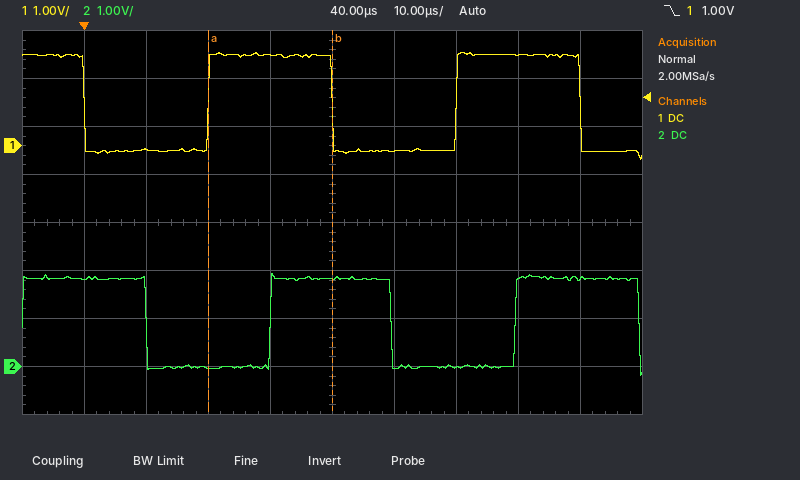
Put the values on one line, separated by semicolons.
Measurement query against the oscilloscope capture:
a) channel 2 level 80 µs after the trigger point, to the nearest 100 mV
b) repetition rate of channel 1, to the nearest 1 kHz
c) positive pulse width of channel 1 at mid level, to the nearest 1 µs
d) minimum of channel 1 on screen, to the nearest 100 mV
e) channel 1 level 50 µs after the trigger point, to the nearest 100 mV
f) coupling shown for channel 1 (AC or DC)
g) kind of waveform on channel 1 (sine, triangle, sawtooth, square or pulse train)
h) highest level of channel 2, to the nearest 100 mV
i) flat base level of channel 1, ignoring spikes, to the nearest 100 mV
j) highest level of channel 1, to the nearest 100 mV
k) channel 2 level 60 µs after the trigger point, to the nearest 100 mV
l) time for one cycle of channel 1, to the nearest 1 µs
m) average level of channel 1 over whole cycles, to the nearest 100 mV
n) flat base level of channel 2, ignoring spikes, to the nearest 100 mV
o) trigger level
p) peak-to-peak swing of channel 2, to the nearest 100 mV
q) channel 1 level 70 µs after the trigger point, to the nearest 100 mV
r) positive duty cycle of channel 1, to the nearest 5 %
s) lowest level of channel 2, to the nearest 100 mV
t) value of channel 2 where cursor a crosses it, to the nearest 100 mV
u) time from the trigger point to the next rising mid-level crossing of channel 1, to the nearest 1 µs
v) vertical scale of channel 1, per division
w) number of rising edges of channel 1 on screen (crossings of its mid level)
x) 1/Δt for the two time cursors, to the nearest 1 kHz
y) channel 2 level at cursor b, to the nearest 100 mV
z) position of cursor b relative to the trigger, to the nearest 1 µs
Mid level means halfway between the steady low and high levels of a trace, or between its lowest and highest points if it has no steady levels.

1.8 V; 25 kHz; 20 µs; -300 mV; -100 mV; DC; square; 1.9 V; -100 mV; 1.9 V; 0.0 V; 40 µs; 900 mV; 0.0 V; 1.00 V; 2.1 V; 1.9 V; 50 %; -200 mV; 0.0 V; 20 µs; 1 V; 2; 50 kHz; 1.8 V; +40 µs
